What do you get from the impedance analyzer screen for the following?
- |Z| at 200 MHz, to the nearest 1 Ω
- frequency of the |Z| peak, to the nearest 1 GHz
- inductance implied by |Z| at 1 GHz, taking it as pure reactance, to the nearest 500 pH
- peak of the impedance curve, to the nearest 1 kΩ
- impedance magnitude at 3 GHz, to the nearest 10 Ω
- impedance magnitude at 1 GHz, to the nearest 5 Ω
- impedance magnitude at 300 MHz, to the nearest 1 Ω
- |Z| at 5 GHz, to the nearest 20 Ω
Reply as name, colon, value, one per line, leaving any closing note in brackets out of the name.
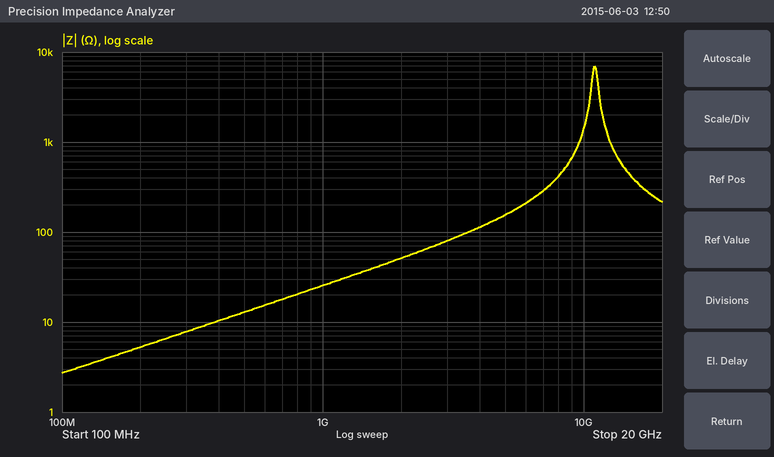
|Z| at 200 MHz, to the nearest 1 Ω: 5 Ω
frequency of the |Z| peak, to the nearest 1 GHz: 11 GHz
inductance implied by |Z| at 1 GHz, taking it as pure reactance, to the nearest 500 pH: 4.0 nH
peak of the impedance curve, to the nearest 1 kΩ: 7 kΩ
impedance magnitude at 3 GHz, to the nearest 10 Ω: 80 Ω
impedance magnitude at 1 GHz, to the nearest 5 Ω: 25 Ω
impedance magnitude at 300 MHz, to the nearest 1 Ω: 8 Ω
|Z| at 5 GHz, to the nearest 20 Ω: 160 Ω
